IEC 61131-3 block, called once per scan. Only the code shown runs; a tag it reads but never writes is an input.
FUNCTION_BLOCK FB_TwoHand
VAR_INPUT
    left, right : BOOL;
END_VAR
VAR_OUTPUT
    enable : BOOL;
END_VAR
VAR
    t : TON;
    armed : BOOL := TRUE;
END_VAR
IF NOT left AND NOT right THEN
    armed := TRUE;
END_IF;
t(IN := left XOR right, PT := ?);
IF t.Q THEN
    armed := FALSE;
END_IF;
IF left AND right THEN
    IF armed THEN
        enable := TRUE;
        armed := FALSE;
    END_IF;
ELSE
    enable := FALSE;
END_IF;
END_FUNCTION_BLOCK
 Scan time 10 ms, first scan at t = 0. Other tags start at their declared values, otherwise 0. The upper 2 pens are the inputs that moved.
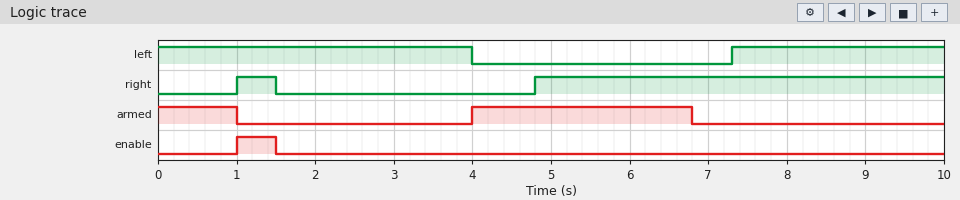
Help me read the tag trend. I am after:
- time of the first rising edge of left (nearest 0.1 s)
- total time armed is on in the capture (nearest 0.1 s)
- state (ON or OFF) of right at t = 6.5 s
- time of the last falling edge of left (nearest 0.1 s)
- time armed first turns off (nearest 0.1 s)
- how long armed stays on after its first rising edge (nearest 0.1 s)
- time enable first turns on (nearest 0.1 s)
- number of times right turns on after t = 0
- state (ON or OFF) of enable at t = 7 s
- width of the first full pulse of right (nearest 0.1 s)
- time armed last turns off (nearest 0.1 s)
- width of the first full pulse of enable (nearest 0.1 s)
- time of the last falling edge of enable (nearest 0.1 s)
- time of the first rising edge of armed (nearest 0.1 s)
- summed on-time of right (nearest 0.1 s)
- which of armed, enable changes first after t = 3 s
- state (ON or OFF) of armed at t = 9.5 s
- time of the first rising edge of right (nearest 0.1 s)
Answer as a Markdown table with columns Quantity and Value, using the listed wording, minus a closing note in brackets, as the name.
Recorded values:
| Quantity | Value |
|---|---|
| time of the first rising edge of left | 7.3 s |
| total time armed is on in the capture | 3.8 s |
| state (ON or OFF) of right at t = 6.5 s | ON |
| time of the last falling edge of left | 4.0 s |
| time armed first turns off | 1.0 s |
| how long armed stays on after its first rising edge | 2.8 s |
| time enable first turns on | 1.0 s |
| number of times right turns on after t = 0 | 2 |
| state (ON or OFF) of enable at t = 7 s | OFF |
| width of the first full pulse of right | 0.5 s |
| time armed last turns off | 6.8 s |
| width of the first full pulse of enable | 0.5 s |
| time of the last falling edge of enable | 1.5 s |
| time of the first rising edge of armed | 4.0 s |
| summed on-time of right | 5.7 s |
| which of armed, enable changes first after t = 3 s | armed |
| state (ON or OFF) of armed at t = 9.5 s | OFF |
| time of the first rising edge of right | 1.0 s |
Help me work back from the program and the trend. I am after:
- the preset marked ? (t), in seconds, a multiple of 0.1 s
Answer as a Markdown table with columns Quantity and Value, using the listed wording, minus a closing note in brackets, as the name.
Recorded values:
| Quantity | Value |
|---|---|
| the preset marked ? (t), in seconds, a multiple of 0.1 s | 2.0 s |
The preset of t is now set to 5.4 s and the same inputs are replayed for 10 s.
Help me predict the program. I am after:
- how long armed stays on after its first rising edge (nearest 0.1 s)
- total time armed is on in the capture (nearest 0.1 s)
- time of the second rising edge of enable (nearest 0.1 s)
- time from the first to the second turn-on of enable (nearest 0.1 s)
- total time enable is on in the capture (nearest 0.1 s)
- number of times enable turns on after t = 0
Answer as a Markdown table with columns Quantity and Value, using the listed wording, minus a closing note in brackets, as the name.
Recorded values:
| Quantity | Value |
|---|---|
| how long armed stays on after its first rising edge | 3.3 s |
| total time armed is on in the capture | 4.3 s |
| time of the second rising edge of enable | 7.3 s |
| time from the first to the second turn-on of enable | 6.3 s |
| total time enable is on in the capture | 3.2 s |
| number of times enable turns on after t = 0 | 2 |
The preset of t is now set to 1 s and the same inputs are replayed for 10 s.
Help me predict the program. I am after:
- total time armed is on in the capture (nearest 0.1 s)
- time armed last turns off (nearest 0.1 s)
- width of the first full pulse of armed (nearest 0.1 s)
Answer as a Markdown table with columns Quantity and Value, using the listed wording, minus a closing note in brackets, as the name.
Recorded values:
| Quantity | Value |
|---|---|
| total time armed is on in the capture | 2.8 s |
| time armed last turns off | 5.8 s |
| width of the first full pulse of armed | 1.8 s |
